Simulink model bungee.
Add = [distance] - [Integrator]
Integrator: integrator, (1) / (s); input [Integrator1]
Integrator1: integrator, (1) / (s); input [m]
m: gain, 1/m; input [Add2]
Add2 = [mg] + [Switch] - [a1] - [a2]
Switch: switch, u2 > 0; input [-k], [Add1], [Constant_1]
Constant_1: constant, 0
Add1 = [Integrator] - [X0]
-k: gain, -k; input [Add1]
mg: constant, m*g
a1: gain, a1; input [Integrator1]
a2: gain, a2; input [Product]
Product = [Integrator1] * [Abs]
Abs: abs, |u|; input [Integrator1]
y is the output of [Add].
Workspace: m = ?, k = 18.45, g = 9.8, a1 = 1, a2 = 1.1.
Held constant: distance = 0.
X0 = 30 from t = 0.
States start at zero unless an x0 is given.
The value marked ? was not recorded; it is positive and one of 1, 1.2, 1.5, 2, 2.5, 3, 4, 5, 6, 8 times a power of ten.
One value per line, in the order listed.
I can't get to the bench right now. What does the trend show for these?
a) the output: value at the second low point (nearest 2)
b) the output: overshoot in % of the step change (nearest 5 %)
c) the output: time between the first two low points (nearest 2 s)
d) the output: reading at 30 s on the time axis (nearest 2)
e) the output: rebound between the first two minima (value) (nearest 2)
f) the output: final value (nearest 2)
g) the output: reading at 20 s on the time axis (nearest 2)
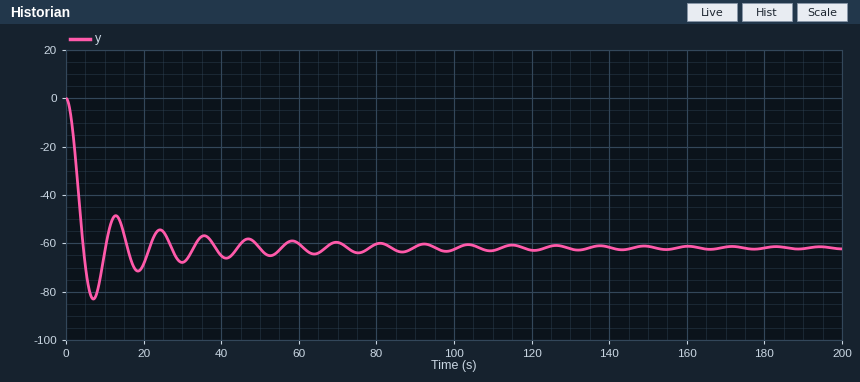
-72
35 %
12 s
-68
-48
-62
-68
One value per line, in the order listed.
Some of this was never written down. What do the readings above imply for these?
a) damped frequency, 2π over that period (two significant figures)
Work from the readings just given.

0.52 rad/s
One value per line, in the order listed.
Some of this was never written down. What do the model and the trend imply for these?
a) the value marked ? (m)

60
